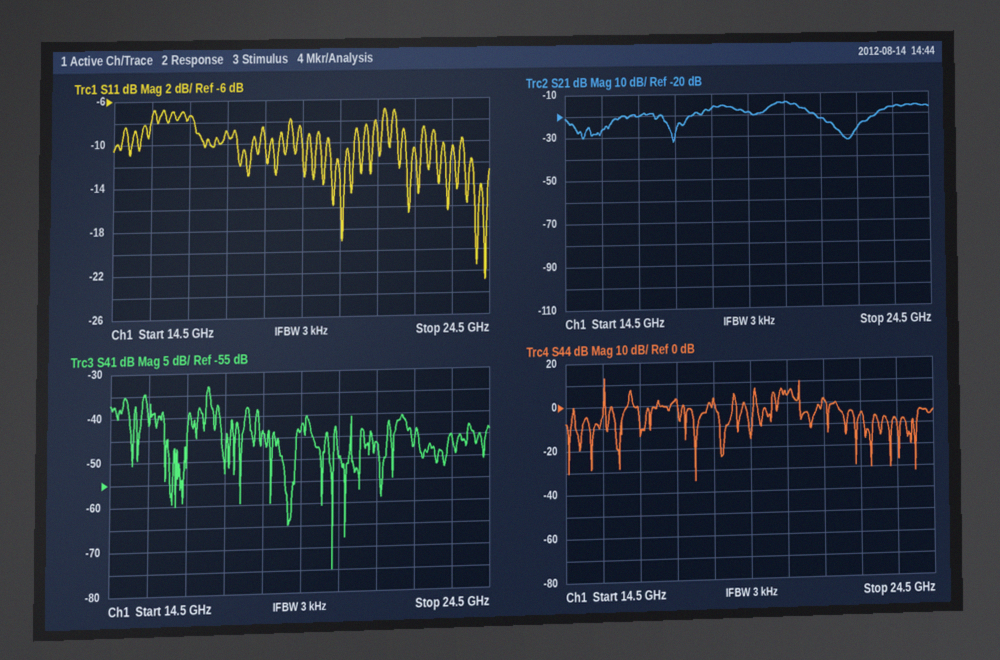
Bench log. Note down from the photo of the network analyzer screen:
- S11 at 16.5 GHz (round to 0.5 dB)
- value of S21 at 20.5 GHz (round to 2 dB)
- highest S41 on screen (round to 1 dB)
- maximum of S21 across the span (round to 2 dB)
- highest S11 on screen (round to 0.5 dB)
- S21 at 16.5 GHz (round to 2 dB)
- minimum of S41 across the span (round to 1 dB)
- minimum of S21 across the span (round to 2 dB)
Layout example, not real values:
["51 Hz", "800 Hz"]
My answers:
["-7.5 dB", "-14 dB", "-33 dB", "-14 dB", "-7.0 dB", "-20 dB", "-75 dB", "-32 dB"]
